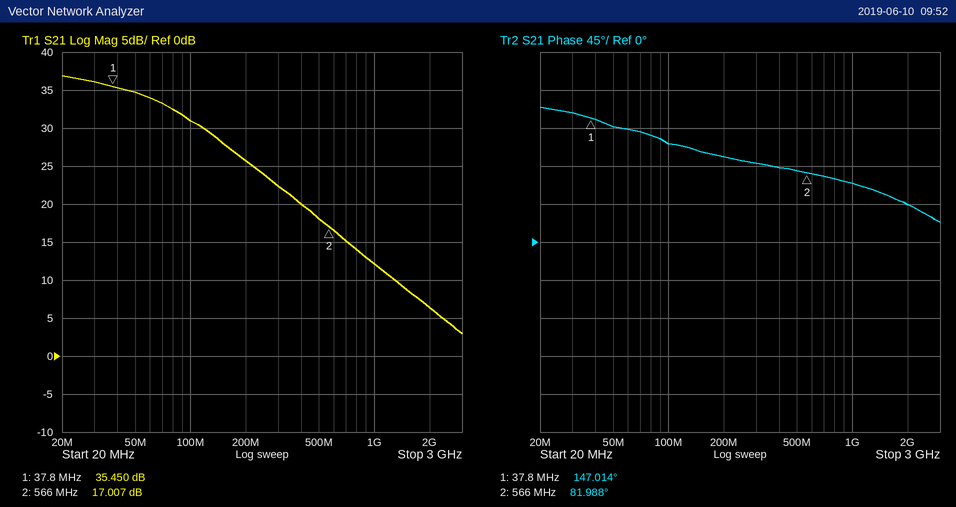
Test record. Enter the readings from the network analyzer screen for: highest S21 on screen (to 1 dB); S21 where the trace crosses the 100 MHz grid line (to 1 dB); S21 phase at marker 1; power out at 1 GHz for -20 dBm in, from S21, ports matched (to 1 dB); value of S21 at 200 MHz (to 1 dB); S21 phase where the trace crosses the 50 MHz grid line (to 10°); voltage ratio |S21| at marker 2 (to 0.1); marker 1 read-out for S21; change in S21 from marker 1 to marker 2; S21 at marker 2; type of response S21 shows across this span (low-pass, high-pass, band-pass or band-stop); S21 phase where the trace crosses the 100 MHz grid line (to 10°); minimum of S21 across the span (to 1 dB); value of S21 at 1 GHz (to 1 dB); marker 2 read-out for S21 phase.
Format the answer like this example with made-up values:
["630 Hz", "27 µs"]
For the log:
["37 dB", "31 dB", "147.014°", "-8 dBm", "26 dB", "140°", "7.1", "35.450 dB", "-18.443 dB", "17.007 dB", "low-pass", "120°", "3 dB", "12 dB", "81.988°"]
